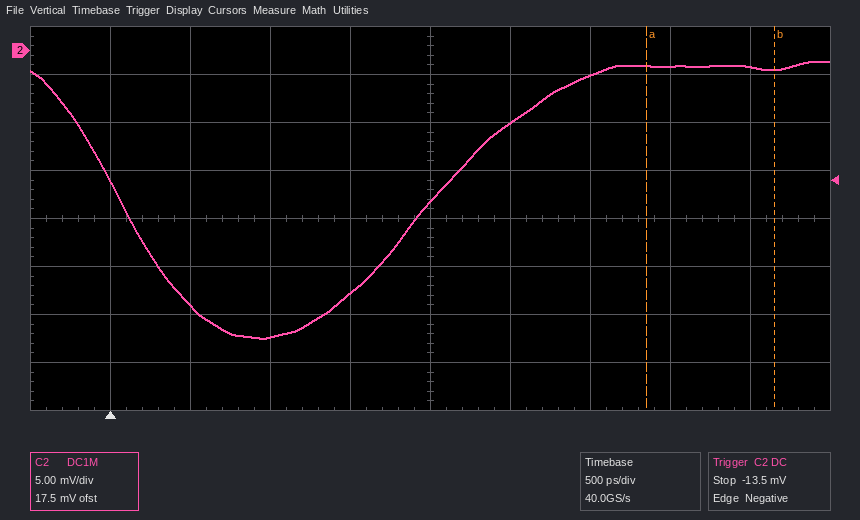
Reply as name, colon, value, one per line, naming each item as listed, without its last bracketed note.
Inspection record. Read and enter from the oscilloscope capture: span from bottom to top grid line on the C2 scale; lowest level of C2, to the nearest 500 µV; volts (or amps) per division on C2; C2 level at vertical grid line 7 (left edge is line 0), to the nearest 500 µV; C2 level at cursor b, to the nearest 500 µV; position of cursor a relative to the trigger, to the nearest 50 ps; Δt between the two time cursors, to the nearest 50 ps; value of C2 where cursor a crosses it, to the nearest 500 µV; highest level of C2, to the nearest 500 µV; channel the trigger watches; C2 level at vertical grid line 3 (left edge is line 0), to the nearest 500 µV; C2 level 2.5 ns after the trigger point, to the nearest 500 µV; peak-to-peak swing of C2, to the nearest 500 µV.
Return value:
span from bottom to top grid line on the C2 scale: 40 mV
lowest level of C2, to the nearest 500 µV: -30.0 mV
volts (or amps) per division on C2: 5 mV
C2 level at vertical grid line 7 (left edge is line 0), to the nearest 500 µV: -2.5 mV
C2 level at cursor b, to the nearest 500 µV: -2.0 mV
position of cursor a relative to the trigger, to the nearest 50 ps: +3.35 ns
Δt between the two time cursors, to the nearest 50 ps: 800 ps
value of C2 where cursor a crosses it, to the nearest 500 µV: -1.5 mV
highest level of C2, to the nearest 500 µV: -1.0 mV
channel the trigger watches: C2
C2 level at vertical grid line 3 (left edge is line 0), to the nearest 500 µV: -30.0 mV
C2 level 2.5 ns after the trigger point, to the nearest 500 µV: -7.5 mV
peak-to-peak swing of C2, to the nearest 500 µV: 29.0 mV
